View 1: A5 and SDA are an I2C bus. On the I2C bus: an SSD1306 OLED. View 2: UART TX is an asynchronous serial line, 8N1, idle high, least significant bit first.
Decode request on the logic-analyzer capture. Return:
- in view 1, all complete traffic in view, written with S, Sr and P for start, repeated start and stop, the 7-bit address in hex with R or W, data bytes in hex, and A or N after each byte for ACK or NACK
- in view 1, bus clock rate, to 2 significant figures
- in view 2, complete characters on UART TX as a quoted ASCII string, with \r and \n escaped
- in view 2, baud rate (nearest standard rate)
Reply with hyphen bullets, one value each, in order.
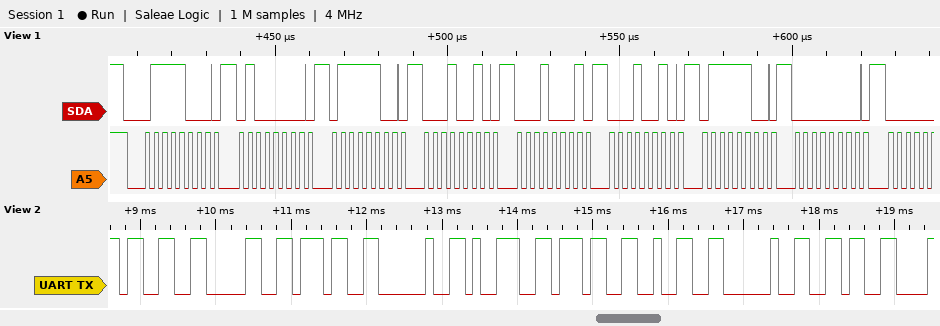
- S 3CW A 40 A 7C A 12 A 11 A 12 A 7C A 00 A
- 400 kHz
- "307 972 6"
- 9600 baud
